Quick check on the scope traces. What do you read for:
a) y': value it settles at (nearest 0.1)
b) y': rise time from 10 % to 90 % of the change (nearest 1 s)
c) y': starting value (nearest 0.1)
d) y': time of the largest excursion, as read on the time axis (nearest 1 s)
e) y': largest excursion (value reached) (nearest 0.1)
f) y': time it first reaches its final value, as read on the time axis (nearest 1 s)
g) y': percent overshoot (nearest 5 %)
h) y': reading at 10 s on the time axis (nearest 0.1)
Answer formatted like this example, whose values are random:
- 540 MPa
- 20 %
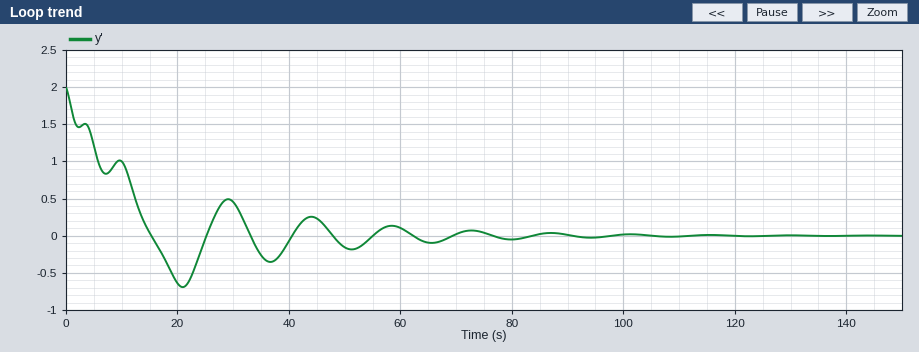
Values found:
- 0.0
- 13 s
- 2.0
- 21 s
- -0.7
- 15 s
- 35 %
- 1.0
